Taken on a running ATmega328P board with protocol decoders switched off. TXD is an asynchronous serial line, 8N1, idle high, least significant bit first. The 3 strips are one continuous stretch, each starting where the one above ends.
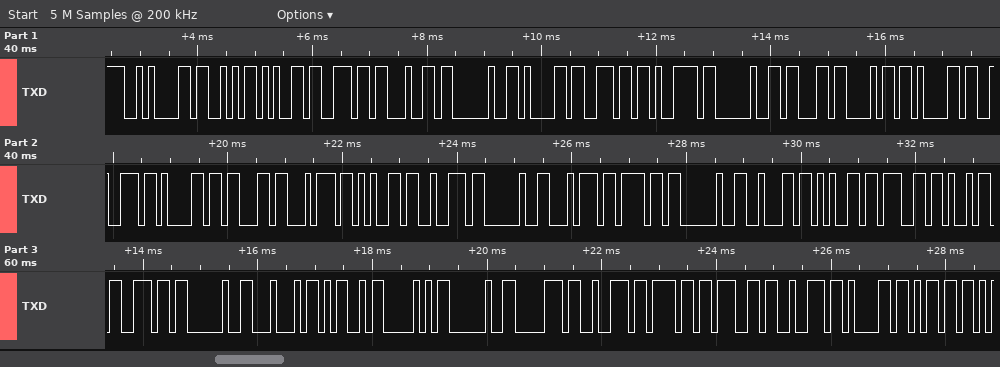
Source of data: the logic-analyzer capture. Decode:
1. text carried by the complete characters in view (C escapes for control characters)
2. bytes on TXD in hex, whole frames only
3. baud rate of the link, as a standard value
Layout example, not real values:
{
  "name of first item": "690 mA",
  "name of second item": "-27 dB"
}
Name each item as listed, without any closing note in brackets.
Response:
{
  "text carried by the complete characters in view": "\"\\nSend any character to begin DMP program\"",
  "bytes on TXD in hex, whole frames only": "0A 53 65 6E 64 20 61 6E 79 20 63 68 61 72 61 63 74 65 72 20 74 6F 20 62 65 67 69 6E 20 44 4D 50 20 70 72 6F 67 72 61 6D",
  "baud rate of the link, as a standard value": "9600 baud"
}
